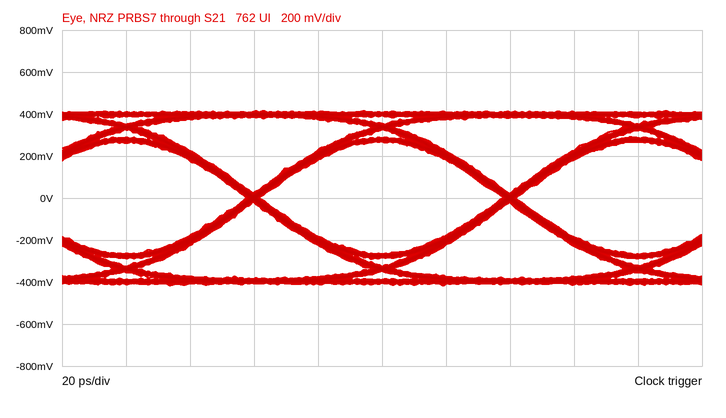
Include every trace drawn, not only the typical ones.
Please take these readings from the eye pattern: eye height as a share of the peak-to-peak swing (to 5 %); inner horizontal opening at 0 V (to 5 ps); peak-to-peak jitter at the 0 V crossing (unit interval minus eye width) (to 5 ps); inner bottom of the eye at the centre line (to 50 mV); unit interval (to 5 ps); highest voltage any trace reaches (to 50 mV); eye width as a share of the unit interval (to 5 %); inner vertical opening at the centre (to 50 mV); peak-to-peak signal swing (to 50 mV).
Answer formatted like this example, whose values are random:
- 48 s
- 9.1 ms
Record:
- 65 %
- 75 ps
- 5 ps
- -250 mV
- 80 ps
- 400 mV
- 95 %
- 550 mV
- 850 mV
